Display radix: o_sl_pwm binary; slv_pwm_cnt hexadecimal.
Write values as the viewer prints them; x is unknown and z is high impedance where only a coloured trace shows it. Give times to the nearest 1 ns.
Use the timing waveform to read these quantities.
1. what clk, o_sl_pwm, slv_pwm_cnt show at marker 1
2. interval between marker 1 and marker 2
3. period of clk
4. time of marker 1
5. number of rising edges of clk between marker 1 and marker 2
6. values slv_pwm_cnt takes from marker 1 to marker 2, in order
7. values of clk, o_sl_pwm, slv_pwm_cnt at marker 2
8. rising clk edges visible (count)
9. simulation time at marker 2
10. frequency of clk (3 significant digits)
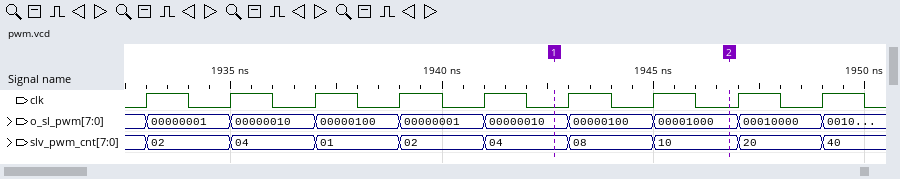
clk=0, o_sl_pwm=00000010, slv_pwm_cnt=04
4 ns
2 ns
1943 ns
2
04, 08, 10
clk=0, o_sl_pwm=00001000, slv_pwm_cnt=10
9
1947 ns
500 MHz
